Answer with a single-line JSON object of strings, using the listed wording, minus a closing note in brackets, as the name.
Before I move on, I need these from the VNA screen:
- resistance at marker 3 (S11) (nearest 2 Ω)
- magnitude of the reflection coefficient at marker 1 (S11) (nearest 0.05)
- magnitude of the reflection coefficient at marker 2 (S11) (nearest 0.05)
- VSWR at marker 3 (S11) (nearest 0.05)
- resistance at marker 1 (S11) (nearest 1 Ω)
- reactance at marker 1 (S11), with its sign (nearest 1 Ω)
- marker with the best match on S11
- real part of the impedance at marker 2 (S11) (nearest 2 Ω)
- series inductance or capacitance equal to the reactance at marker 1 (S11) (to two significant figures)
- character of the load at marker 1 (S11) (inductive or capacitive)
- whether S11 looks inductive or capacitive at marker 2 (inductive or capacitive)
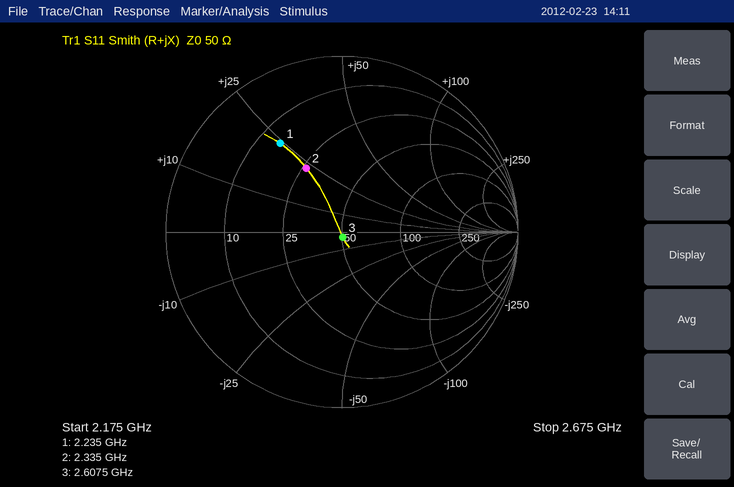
{"resistance at marker 3 (S11)": "50 Ω", "magnitude of the reflection coefficient at marker 1 (S11)": "0.60", "magnitude of the reflection coefficient at marker 2 (S11)": "0.40", "VSWR at marker 3 (S11)": "1.05", "resistance at marker 1 (S11)": "15 Ω", "reactance at marker 1 (S11), with its sign": "+24 Ω", "marker with the best match on S11": "marker 3", "real part of the impedance at marker 2 (S11)": "26 Ω", "series inductance or capacitance equal to the reactance at marker 1 (S11)": "1.7 nH", "character of the load at marker 1 (S11)": "inductive", "whether S11 looks inductive or capacitive at marker 2": "inductive"}
